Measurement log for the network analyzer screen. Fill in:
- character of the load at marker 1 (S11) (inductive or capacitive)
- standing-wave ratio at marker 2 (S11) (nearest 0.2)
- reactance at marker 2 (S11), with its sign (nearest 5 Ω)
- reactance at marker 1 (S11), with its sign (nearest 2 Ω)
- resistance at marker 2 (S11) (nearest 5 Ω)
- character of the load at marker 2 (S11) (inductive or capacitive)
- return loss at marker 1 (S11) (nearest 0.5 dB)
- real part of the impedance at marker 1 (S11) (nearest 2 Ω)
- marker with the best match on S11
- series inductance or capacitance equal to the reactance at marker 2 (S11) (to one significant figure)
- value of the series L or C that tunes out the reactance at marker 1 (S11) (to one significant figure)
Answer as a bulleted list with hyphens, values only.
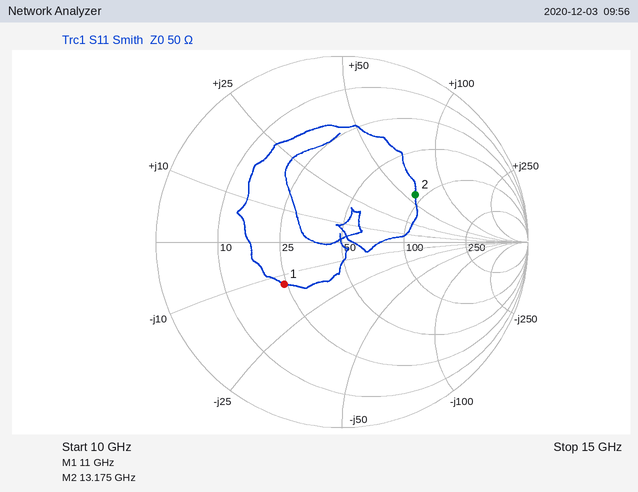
- capacitive
- 2.8
- +60 Ω
- -12 Ω
- 90 Ω
- inductive
- 8.5 dB
- 24 Ω
- marker 1
- 700 pH
- 200 pH
